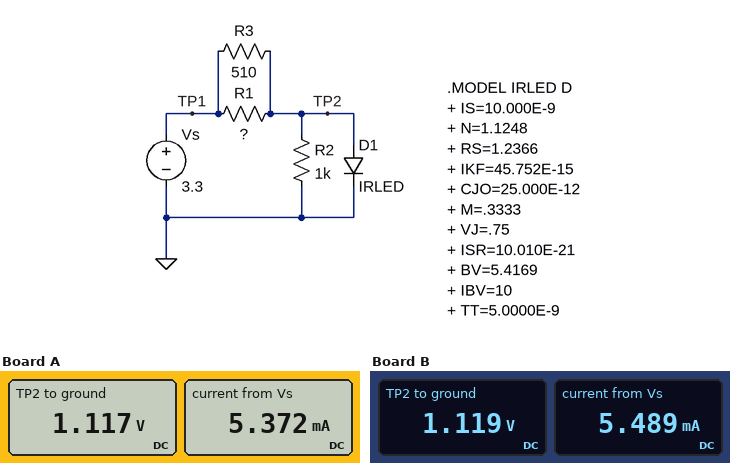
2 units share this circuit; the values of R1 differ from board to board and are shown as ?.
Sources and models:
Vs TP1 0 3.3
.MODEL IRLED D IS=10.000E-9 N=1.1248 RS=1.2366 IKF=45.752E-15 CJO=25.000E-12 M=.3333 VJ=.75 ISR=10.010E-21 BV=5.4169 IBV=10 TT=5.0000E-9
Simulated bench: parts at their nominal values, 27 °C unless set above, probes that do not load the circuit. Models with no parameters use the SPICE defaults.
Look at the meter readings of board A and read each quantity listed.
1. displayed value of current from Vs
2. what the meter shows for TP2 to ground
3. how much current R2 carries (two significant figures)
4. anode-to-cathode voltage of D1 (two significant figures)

5.372 mA
1.117 V
1.1 mA
1.1 V
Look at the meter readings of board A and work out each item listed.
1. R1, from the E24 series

2 kΩ
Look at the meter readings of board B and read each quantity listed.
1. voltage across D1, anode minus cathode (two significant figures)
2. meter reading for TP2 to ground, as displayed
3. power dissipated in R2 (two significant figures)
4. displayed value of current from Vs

1.1 V
1.119 V
1.3 mW
5.489 mA
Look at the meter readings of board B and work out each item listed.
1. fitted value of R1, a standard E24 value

1.8 kΩ
